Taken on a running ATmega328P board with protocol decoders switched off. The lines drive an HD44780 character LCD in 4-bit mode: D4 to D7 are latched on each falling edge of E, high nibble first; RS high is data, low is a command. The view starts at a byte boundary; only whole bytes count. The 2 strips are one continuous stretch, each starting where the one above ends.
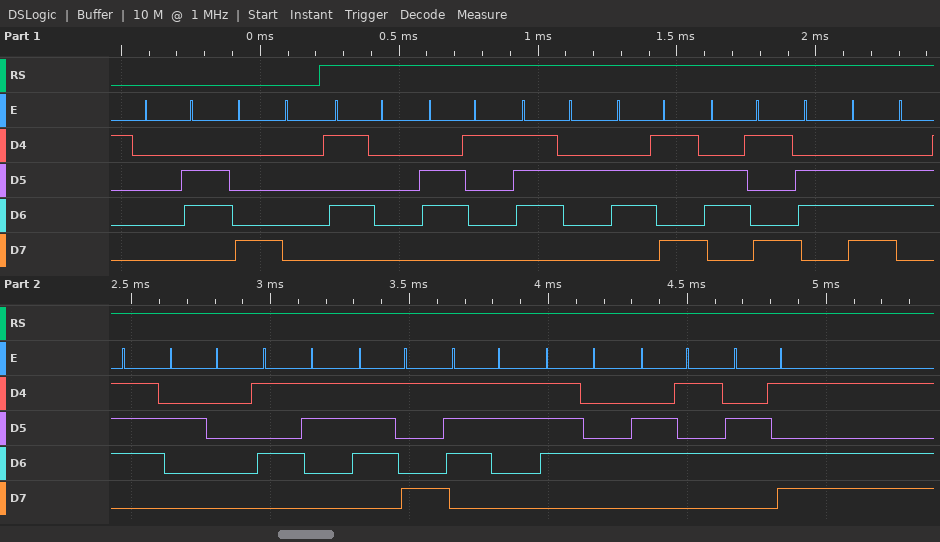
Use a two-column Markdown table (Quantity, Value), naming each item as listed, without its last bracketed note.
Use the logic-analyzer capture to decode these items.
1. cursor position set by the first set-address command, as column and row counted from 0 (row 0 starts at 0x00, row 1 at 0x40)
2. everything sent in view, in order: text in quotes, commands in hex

| Quantity | Value |
|---|---|
| cursor position set by the first set-address command, as column and row counted from 0 | column 0, row 0 |
| everything sent in view, in order: text in quotes, commands in hex | 0x06 0x80 "Parking System" |
